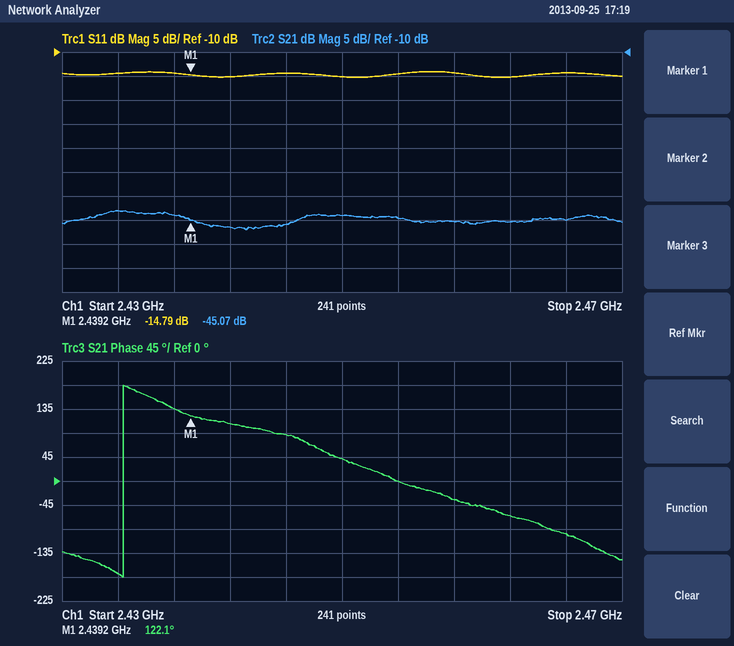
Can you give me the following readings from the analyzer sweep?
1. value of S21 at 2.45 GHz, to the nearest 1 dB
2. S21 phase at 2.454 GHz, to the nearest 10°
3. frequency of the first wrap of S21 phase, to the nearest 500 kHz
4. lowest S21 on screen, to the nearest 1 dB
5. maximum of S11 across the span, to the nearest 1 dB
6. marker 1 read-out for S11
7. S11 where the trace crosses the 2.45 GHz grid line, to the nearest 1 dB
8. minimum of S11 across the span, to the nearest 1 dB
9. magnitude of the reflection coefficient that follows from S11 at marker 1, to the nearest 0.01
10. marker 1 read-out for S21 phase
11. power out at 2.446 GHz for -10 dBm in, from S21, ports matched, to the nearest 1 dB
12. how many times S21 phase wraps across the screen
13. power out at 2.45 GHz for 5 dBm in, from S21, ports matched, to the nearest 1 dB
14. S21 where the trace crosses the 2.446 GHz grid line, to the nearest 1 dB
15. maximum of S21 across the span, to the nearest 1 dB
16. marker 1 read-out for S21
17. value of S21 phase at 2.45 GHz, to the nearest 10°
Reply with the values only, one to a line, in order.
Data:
-44 dB
0°
2.4345 GHz
-47 dB
-14 dB
-14.79 dB
-15 dB
-15 dB
0.18
122.1°
-56 dBm
1
-39 dBm
-46 dB
-43 dB
-45.07 dB
40°
